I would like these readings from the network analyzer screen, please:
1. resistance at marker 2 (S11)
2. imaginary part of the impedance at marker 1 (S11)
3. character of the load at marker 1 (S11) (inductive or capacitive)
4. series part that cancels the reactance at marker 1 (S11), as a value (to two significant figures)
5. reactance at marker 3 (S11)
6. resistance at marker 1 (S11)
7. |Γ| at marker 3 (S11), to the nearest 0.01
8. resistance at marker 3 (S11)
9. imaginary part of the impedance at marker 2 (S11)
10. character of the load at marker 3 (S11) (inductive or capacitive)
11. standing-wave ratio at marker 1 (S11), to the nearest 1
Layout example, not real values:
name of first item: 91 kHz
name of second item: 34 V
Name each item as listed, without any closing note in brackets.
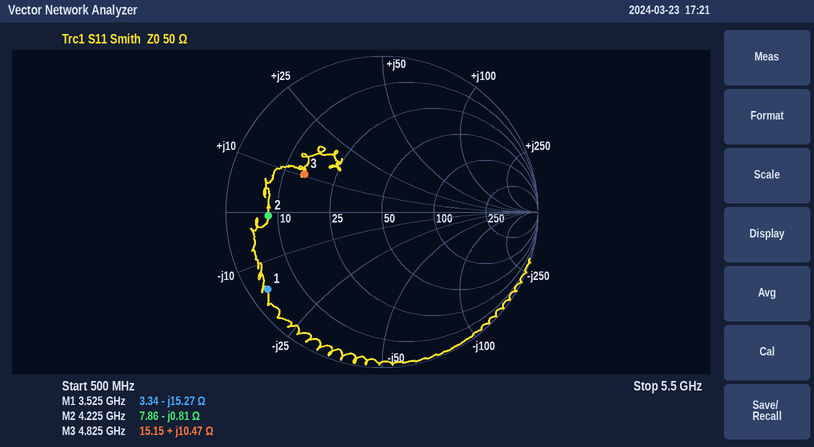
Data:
resistance at marker 2: 7.86 Ω
imaginary part of the impedance at marker 1: -15.27 Ω
character of the load at marker 1 (S11): capacitive
series part that cancels the reactance at marker 1 (S11), as a value: 690 pH
reactance at marker 3: +10.47 Ω
resistance at marker 1: 3.34 Ω
|Γ| at marker 3 (S11), to the nearest 0.01: 0.55
resistance at marker 3: 15.15 Ω
imaginary part of the impedance at marker 2: -0.81 Ω
character of the load at marker 3 (S11): inductive
standing-wave ratio at marker 1 (S11), to the nearest 1: 16
